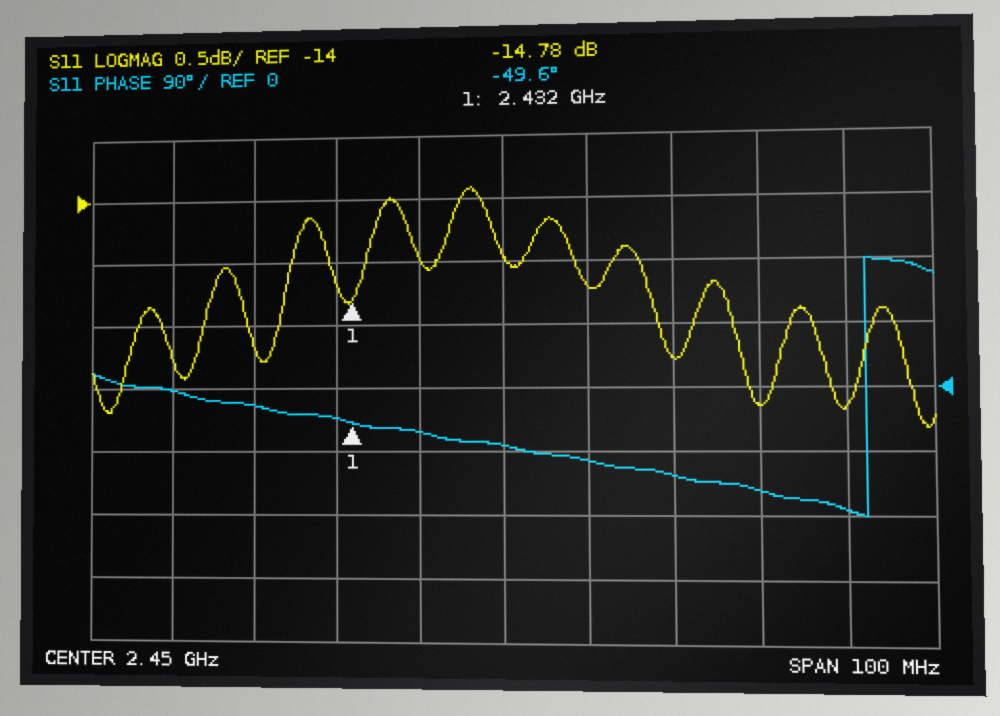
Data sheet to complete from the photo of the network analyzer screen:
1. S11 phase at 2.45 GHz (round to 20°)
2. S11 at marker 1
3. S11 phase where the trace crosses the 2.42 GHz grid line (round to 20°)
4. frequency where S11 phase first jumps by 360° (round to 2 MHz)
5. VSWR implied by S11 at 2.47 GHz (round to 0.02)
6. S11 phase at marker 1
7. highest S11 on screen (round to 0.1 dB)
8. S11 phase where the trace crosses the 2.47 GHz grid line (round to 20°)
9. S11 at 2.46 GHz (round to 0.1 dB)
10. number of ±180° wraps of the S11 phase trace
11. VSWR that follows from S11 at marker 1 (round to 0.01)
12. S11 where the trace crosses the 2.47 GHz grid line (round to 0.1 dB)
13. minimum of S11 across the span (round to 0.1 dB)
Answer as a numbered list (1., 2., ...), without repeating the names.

1. -80°
2. -14.78 dB
3. -20°
4. 2.492 GHz
5. 1.42
6. -49.6°
7. -13.9 dB
8. -120°
9. -14.7 dB
10. 1
11. 1.45
12. -15.3 dB
13. -15.8 dB
